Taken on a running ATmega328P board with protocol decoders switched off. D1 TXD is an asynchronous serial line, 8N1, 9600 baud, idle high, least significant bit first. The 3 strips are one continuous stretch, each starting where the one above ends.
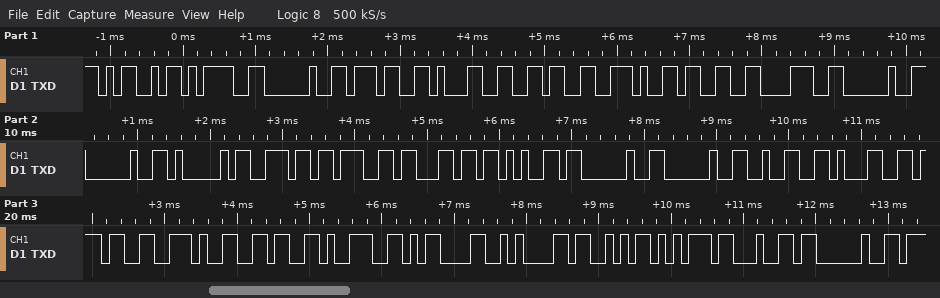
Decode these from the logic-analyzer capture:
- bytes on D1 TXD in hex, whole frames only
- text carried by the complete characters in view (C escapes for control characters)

4D 3D 20 37 31 36 2E 33 38 20 20 41 6E 67 6C 65 20 20 32 31 37 2E 36 39 0D 0A 53 75 64 20
"M= 716.38  Angle  217.69\r\nSud "
